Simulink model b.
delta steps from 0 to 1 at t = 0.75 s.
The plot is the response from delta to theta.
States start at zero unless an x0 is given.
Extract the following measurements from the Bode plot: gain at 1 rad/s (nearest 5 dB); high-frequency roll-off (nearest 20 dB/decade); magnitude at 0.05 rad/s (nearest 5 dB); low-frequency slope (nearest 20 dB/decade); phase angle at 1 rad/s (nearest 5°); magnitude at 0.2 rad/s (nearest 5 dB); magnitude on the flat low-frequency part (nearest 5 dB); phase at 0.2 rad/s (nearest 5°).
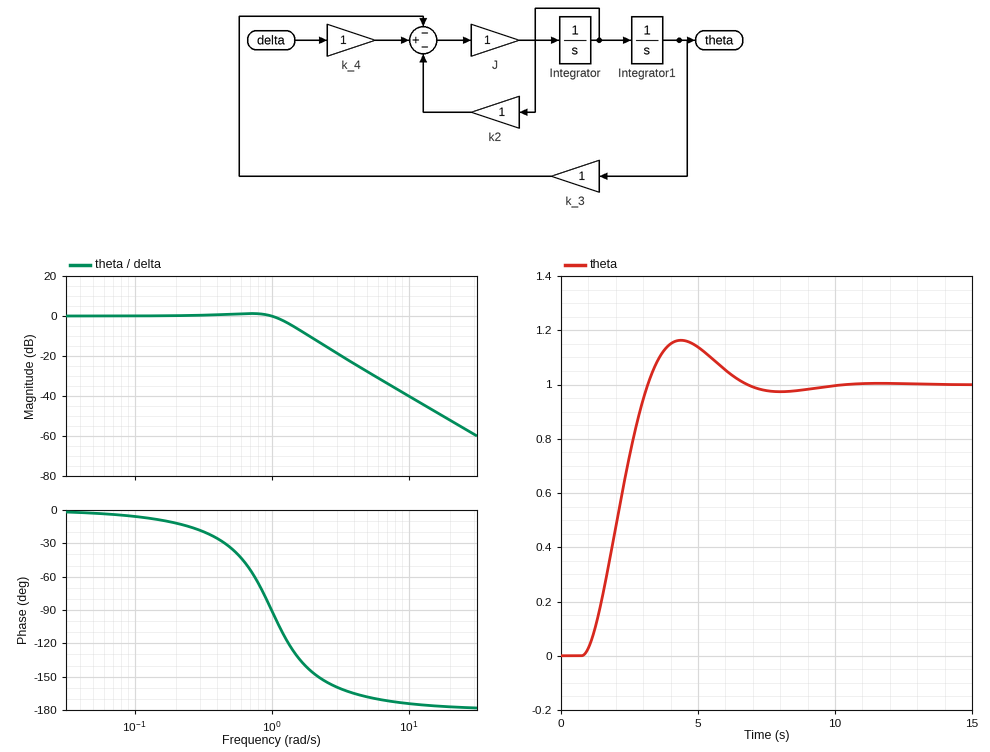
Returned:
0 dB
-40 dB/decade
0 dB
0 dB/decade
-90°
0 dB
0 dB
-10°
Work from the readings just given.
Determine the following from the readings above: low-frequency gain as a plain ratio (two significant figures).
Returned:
1.0
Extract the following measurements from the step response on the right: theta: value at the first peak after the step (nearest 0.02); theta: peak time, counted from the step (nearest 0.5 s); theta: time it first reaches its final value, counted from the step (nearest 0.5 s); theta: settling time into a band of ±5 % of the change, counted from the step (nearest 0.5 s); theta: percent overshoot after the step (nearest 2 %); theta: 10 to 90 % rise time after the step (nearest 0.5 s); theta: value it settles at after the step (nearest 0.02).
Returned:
1.16
3.5 s
2.5 s
5.5 s
16 %
1.5 s
1.00
